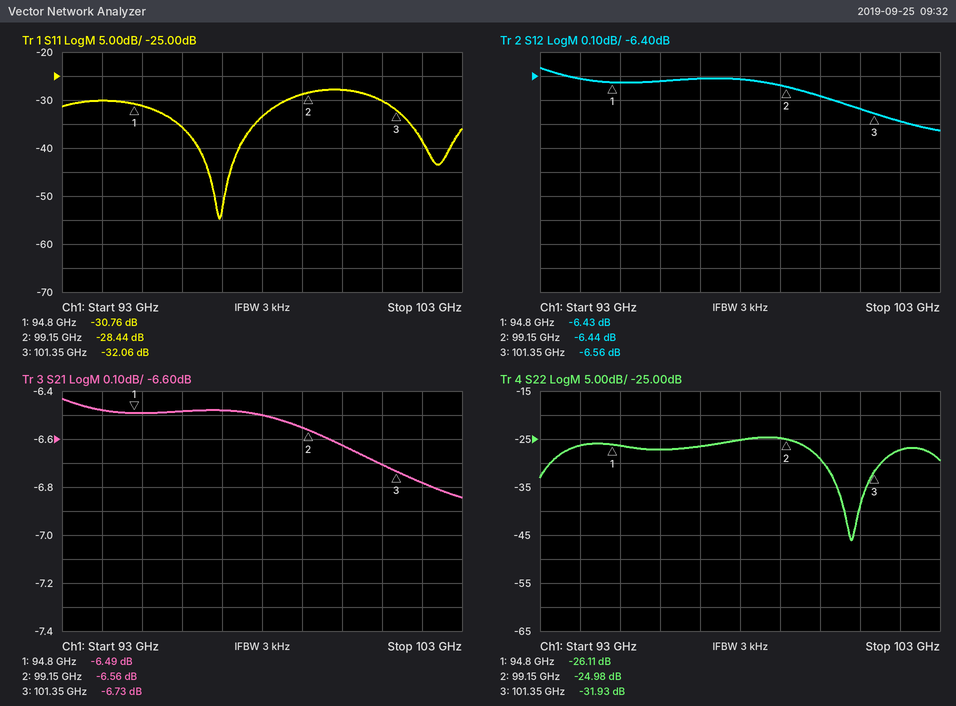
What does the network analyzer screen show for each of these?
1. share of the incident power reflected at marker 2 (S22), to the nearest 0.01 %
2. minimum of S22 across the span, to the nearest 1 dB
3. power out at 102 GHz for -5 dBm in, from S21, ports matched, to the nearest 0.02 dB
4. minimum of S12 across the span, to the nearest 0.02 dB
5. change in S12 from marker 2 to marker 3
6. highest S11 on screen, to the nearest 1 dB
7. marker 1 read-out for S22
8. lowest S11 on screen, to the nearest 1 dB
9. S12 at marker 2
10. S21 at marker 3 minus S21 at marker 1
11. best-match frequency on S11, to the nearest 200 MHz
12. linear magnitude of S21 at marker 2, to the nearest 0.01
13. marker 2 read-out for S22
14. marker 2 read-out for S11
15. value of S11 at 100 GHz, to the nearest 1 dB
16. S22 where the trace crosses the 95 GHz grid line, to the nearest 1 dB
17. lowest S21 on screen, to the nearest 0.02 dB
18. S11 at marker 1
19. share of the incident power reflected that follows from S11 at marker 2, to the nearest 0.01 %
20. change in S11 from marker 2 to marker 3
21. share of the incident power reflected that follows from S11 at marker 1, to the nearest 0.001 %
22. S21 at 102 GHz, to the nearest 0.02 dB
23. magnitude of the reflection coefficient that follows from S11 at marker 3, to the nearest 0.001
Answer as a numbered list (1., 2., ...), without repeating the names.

1. 0.32 %
2. -46 dB
3. -11.78 dBm
4. -6.62 dB
5. -0.12 dB
6. -28 dB
7. -26.11 dB
8. -55 dB
9. -6.44 dB
10. -0.24 dB
11. 97.0 GHz
12. 0.47
13. -24.98 dB
14. -28.44 dB
15. -28 dB
16. -26 dB
17. -6.84 dB
18. -30.76 dB
19. 0.14 %
20. -3.62 dB
21. 0.084 %
22. -6.78 dB
23. 0.025
